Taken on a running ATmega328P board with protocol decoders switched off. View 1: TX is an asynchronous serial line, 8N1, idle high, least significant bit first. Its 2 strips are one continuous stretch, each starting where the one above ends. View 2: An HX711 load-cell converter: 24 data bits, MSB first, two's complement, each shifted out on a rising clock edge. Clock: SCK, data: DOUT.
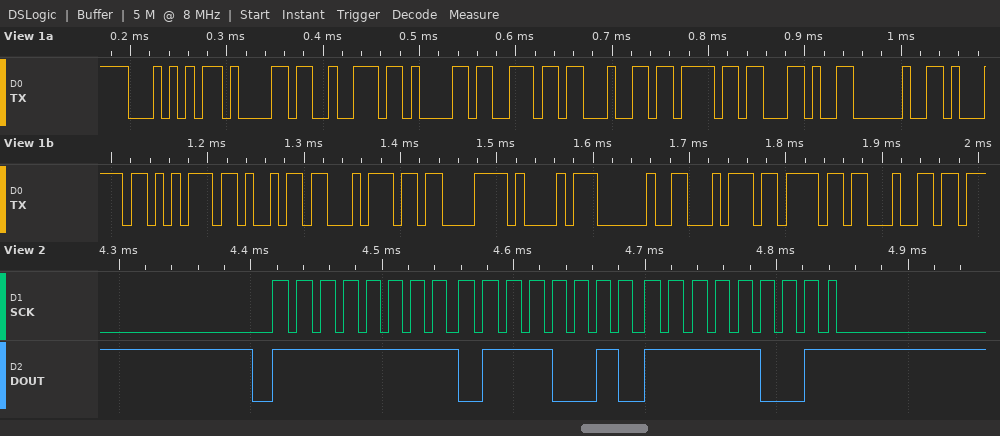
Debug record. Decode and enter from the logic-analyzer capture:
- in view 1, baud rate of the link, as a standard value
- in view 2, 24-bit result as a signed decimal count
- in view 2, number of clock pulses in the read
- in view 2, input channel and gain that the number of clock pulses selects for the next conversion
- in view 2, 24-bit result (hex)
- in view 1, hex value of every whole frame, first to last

115200 baud
-36103
25
channel A, gain 128
0xFF72F9
54 61 72 61 6E 64 6F 2C 20 71 75 69 74 C3 A1 20 74 6F 64
